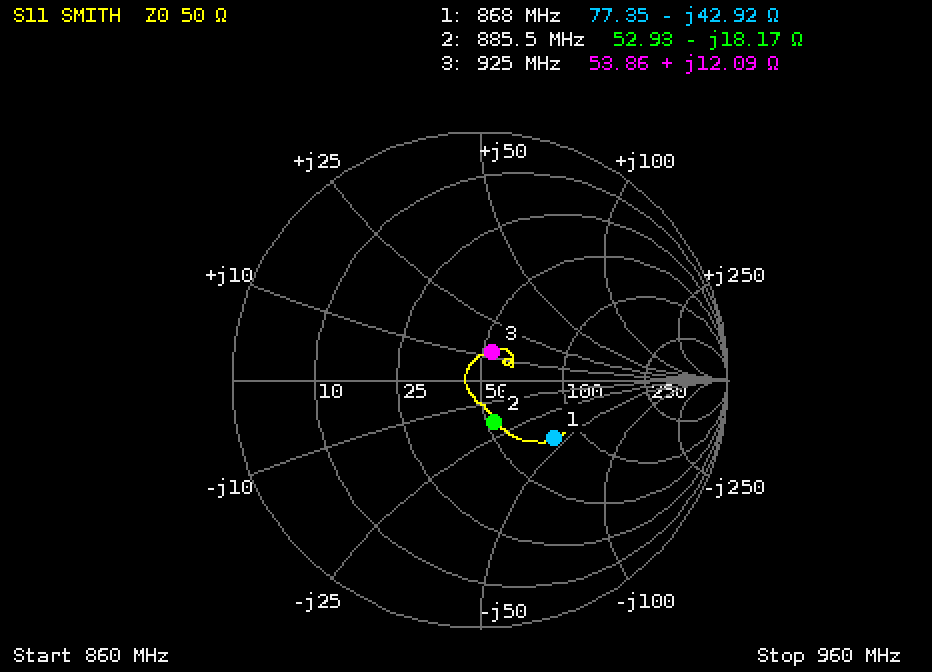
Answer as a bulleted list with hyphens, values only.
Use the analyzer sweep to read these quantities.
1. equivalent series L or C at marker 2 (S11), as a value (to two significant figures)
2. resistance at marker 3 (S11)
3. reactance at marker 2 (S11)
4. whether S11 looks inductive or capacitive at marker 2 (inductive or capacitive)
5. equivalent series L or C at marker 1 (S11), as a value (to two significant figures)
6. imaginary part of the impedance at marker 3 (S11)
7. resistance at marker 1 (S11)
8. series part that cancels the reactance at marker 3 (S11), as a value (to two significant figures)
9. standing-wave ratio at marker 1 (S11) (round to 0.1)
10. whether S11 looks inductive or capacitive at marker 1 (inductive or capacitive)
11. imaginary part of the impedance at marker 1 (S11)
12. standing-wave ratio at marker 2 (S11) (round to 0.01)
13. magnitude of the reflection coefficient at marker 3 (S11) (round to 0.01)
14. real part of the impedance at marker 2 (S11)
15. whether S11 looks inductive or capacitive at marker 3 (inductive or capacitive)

- 9.9 pF
- 53.86 Ω
- -18.17 Ω
- capacitive
- 4.3 pF
- +12.09 Ω
- 77.35 Ω
- 14 pF
- 2.2
- capacitive
- -42.92 Ω
- 1.43
- 0.12
- 52.93 Ω
- inductive
